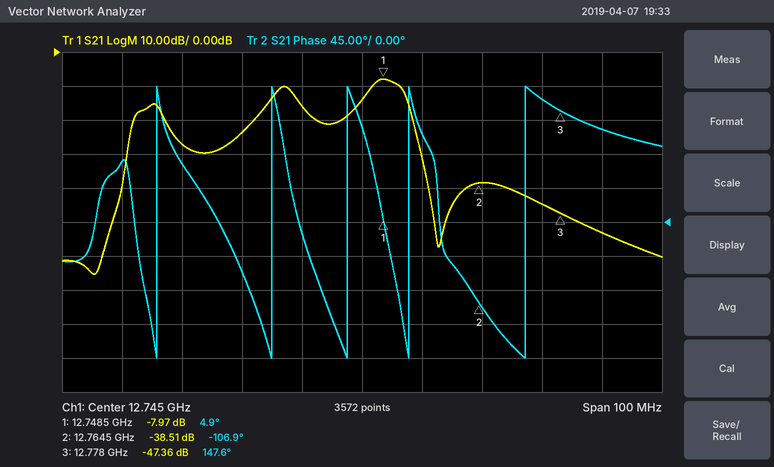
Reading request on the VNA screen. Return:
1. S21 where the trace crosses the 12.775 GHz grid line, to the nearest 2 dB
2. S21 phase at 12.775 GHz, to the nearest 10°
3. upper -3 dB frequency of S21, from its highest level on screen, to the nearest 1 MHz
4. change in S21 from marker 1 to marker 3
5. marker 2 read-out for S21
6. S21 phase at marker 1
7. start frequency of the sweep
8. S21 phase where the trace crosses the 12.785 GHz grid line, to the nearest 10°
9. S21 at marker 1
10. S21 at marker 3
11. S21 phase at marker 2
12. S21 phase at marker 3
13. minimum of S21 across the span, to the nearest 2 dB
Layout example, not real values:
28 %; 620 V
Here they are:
-44 dB; 160°; 12.752 GHz; -39.39 dB; -38.51 dB; 4.9°; 12.695 GHz; 120°; -7.97 dB; -47.36 dB; -106.9°; 147.6°; -66 dB
